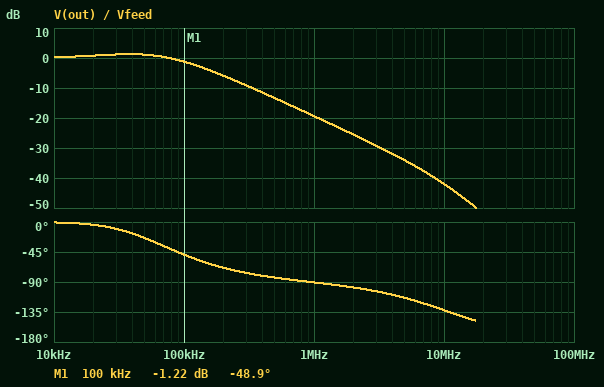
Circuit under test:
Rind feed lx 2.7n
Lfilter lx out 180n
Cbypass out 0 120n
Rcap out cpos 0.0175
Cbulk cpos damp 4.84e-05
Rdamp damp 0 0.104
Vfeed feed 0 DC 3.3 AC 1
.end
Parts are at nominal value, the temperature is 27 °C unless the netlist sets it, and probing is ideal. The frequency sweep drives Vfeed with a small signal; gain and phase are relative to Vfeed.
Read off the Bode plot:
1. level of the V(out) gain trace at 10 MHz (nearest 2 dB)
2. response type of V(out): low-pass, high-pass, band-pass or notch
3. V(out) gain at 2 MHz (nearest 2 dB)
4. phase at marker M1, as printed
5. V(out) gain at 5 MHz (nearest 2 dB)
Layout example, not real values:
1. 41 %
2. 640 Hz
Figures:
1. -42 dB
2. low-pass
3. -26 dB
4. -48.9 deg
5. -34 dB
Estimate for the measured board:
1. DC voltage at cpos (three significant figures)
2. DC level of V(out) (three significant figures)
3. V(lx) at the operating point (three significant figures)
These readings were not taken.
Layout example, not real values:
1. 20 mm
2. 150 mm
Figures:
1. 3.30 V
2. 3.30 V
3. 3.30 V
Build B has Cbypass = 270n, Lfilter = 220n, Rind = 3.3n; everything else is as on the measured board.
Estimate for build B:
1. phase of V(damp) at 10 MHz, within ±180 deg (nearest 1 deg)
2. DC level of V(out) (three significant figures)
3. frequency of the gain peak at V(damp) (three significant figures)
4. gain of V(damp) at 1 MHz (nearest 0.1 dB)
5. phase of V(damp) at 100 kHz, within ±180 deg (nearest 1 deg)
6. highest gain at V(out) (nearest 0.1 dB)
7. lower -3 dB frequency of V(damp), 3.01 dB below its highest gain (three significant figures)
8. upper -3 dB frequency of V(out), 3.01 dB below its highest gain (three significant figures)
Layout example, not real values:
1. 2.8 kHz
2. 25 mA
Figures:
1. -154 deg
2. 3.30 V
3. 49.1 kHz
4. -22.6 dB
5. -42 deg
6. 1.5 dB
7. 21.8 kHz
8. 92.2 kHz
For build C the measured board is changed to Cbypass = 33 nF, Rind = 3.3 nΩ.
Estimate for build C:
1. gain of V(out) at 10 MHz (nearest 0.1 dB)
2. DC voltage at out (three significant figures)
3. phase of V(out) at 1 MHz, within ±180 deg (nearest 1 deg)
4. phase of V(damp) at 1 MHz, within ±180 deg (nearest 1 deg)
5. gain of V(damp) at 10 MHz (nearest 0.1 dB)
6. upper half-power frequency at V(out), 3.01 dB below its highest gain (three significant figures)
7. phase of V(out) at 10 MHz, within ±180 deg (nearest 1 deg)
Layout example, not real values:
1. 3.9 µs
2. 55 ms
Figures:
1. -39.6 dB
2. 3.30 V
3. -87 deg
4. -85 deg
5. -41.0 dB
6. 109 kHz
7. -104 deg
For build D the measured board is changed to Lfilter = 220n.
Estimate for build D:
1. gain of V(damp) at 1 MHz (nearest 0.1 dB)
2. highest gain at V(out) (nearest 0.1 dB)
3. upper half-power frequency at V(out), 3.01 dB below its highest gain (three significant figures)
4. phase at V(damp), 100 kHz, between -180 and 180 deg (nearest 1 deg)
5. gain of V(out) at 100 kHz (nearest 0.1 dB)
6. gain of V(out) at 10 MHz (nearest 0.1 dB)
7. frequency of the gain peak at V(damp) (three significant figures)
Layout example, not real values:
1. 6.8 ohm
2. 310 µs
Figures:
1. -22.5 dB
2. 1.5 dB
3. 91.7 kHz
4. -41 deg
5. -2.1 dB
6. -43.7 dB
7. 48.9 kHz
